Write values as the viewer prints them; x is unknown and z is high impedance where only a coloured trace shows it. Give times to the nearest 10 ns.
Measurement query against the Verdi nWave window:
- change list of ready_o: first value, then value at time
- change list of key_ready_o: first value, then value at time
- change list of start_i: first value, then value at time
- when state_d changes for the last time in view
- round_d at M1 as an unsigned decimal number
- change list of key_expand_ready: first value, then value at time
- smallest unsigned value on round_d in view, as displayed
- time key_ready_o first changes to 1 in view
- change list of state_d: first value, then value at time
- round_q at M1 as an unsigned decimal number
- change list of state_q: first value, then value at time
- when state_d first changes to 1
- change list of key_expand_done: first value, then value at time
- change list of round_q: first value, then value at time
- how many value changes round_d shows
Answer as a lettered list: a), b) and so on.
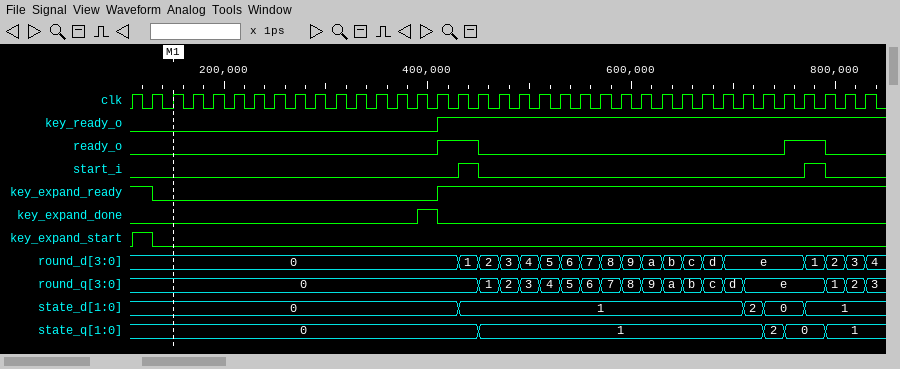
a) 0, 1 at 410 ns, 0 at 450 ns, 1 at 750 ns, 0 at 790 ns
b) 0, 1 at 410 ns
c) 0, 1 at 430 ns, 0 at 450 ns, 1 at 770 ns, 0 at 790 ns
d) 770 ns
e) 0
f) 1, 0 at 130 ns, 1 at 410 ns
g) 0
h) 410 ns
i) 0, 1 at 430 ns, 2 at 710 ns, 0 at 730 ns, 1 at 770 ns
j) 0
k) 0, 1 at 450 ns, 2 at 730 ns, 0 at 750 ns, 1 at 790 ns
l) 430 ns
m) 0, 1 at 390 ns, 0 at 410 ns
n) 0, 1 at 450 ns, 2 at 470 ns, 3 at 490 ns, 4 at 510 ns, 5 at 530 ns, 6 at 550 ns, 7 at 570 ns, 8 at 590 ns, 9 at 610 ns, a at 630 ns, b at 650 ns, c at 670 ns, d at 690 ns, e at 710 ns, 1 at 790 ns, 2 at 810 ns, 3 at 830 ns
o) 18
